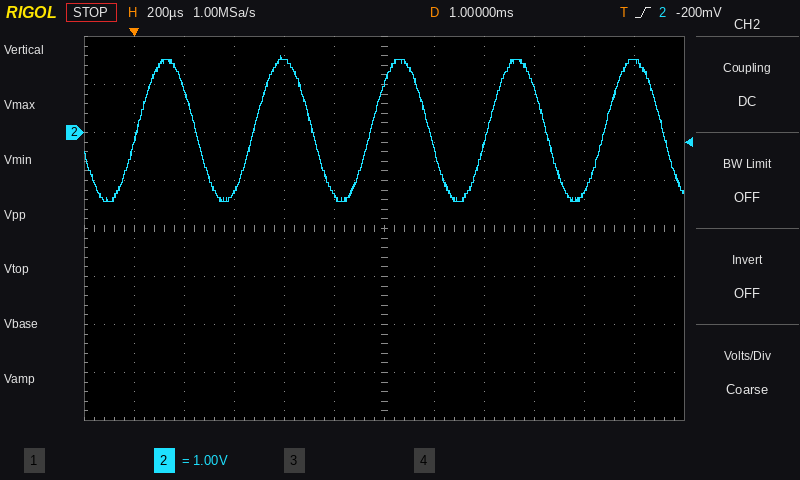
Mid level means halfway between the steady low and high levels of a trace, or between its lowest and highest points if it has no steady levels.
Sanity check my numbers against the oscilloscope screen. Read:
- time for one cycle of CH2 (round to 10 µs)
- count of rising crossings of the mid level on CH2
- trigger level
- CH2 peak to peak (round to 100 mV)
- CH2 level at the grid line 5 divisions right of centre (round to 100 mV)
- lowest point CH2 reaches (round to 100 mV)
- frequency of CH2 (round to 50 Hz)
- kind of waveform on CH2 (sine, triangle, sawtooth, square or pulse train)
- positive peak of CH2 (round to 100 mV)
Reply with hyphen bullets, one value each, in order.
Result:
- 470 µs
- 5
- -200 mV
- 3.0 V
- 1.5 V
- -1.4 V
- 2.15 kHz
- sine
- 1.6 V
